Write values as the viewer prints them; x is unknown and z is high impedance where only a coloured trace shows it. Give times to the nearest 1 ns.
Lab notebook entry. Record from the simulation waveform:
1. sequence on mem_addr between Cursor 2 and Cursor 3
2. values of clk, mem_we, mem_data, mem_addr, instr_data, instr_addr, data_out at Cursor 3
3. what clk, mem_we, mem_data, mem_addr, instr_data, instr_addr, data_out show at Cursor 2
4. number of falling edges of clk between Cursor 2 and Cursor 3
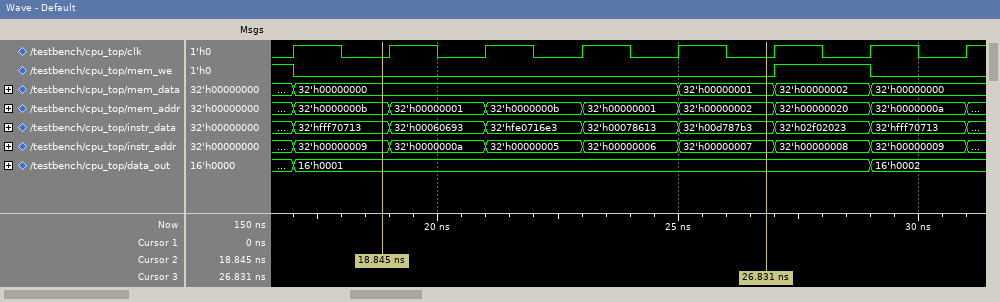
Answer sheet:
32'h0000000b, 32'h00000001, 32'h0000000b, 32'h00000001, 32'h00000002
clk=0, mem_we=0, mem_data=32'h00000001, mem_addr=32'h00000002, instr_data=32'h00d787b3, instr_addr=32'h00000007, data_out=16'h0001
clk=0, mem_we=0, mem_data=32'h00000000, mem_addr=32'h0000000b, instr_data=32'hfff70713, instr_addr=32'h00000009, data_out=16'h0001
4
